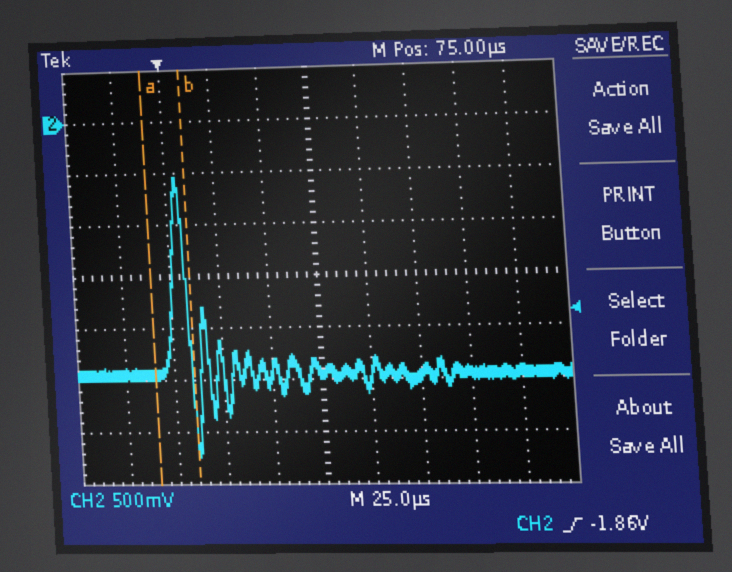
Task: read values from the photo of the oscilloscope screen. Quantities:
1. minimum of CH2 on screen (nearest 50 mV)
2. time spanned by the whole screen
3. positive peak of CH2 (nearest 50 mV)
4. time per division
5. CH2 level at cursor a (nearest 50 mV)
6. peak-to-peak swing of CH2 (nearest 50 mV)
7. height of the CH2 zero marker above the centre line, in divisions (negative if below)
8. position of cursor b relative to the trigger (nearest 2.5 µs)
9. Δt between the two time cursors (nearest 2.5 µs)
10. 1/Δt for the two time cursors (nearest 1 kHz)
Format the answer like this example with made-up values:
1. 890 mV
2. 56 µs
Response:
1. -3.25 V
2. 250 µs
3. -550 mV
4. 25 µs
5. -2.45 V
6. 2.70 V
7. +3.0 div
8. +10.0 µs
9. 20.0 µs
10. 50 kHz
